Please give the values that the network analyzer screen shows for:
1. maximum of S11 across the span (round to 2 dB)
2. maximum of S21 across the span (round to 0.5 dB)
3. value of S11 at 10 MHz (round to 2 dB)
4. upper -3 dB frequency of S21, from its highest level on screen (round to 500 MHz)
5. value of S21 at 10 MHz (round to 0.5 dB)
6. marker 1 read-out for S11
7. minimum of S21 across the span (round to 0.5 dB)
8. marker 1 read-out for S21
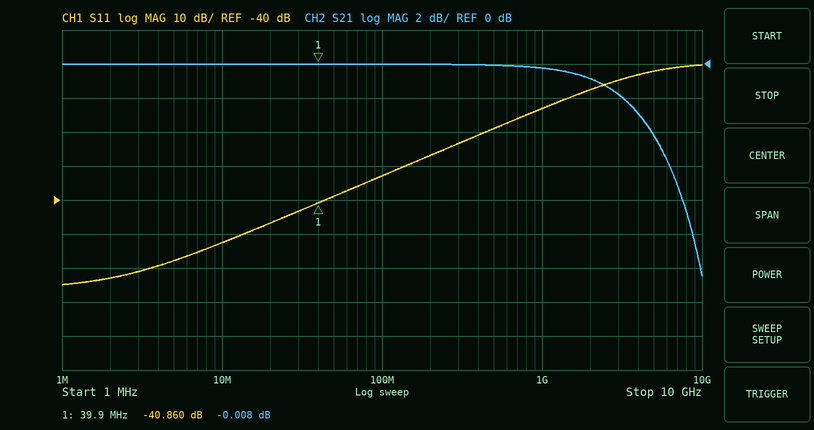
0 dB
0.0 dB
-52 dB
4.0 GHz
0.0 dB
-40.860 dB
-12.5 dB
-0.008 dB
